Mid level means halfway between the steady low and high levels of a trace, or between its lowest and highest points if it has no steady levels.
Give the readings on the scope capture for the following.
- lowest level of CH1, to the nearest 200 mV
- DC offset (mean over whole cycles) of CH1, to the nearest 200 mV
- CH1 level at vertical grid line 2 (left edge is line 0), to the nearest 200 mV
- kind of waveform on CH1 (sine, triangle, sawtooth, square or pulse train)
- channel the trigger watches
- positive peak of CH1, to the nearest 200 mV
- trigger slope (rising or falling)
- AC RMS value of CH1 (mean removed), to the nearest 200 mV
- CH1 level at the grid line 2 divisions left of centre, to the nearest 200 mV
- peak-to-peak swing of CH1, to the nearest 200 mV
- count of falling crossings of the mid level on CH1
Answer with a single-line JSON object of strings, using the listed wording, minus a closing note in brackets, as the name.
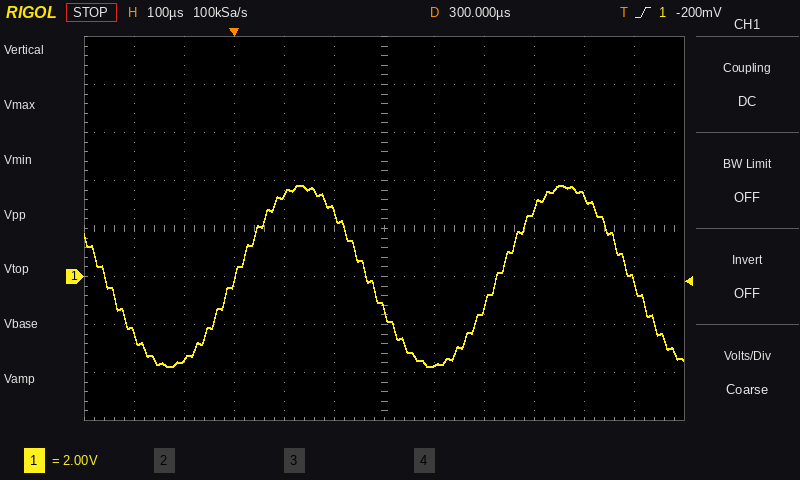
{"lowest level of CH1, to the nearest 200 mV": "-3.8 V", "DC offset (mean over whole cycles) of CH1, to the nearest 200 mV": "0.0 V", "CH1 level at vertical grid line 2 (left edge is line 0), to the nearest 200 mV": "-3.4 V", "kind of waveform on CH1": "sine", "channel the trigger watches": "CH1", "positive peak of CH1, to the nearest 200 mV": "3.8 V", "trigger slope": "rising", "AC RMS value of CH1 (mean removed), to the nearest 200 mV": "2.6 V", "CH1 level at the grid line 2 divisions left of centre, to the nearest 200 mV": "3.4 V", "peak-to-peak swing of CH1, to the nearest 200 mV": "7.6 V", "count of falling crossings of the mid level on CH1": "3"}
